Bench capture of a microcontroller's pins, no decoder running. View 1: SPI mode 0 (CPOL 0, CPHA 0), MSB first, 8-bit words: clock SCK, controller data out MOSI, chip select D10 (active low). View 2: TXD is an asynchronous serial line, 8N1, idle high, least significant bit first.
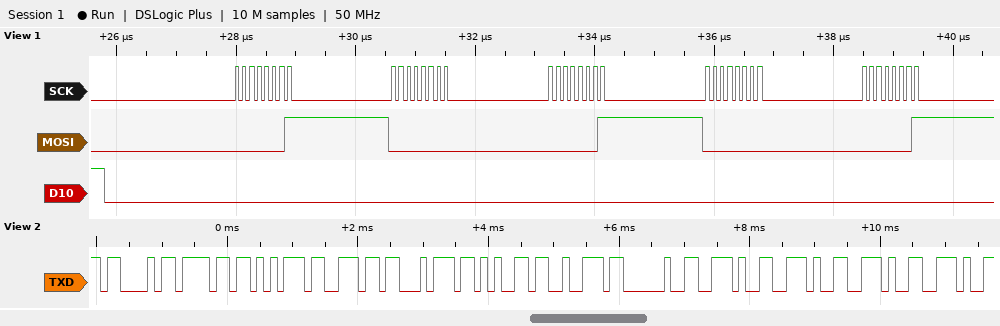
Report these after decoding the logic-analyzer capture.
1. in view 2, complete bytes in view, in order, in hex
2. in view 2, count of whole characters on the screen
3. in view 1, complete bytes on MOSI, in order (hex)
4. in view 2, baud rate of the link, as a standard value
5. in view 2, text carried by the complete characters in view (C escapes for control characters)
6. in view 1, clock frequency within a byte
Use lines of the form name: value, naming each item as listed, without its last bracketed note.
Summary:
in view 2, complete bytes in view, in order, in hex: 0x43 0x6F 0x75 0x6E 0x74 0x65 0x72 0x20 0x2E 0x2E 0x2E 0x2E
in view 2, count of whole characters on the screen: 12
in view 1, complete bytes on MOSI, in order: 01 00 01 00 01
in view 2, baud rate of the link, as a standard value: 9600 baud
in view 2, text carried by the complete characters in view: "Counter ...."
in view 1, clock frequency within a byte: 8 MHz
